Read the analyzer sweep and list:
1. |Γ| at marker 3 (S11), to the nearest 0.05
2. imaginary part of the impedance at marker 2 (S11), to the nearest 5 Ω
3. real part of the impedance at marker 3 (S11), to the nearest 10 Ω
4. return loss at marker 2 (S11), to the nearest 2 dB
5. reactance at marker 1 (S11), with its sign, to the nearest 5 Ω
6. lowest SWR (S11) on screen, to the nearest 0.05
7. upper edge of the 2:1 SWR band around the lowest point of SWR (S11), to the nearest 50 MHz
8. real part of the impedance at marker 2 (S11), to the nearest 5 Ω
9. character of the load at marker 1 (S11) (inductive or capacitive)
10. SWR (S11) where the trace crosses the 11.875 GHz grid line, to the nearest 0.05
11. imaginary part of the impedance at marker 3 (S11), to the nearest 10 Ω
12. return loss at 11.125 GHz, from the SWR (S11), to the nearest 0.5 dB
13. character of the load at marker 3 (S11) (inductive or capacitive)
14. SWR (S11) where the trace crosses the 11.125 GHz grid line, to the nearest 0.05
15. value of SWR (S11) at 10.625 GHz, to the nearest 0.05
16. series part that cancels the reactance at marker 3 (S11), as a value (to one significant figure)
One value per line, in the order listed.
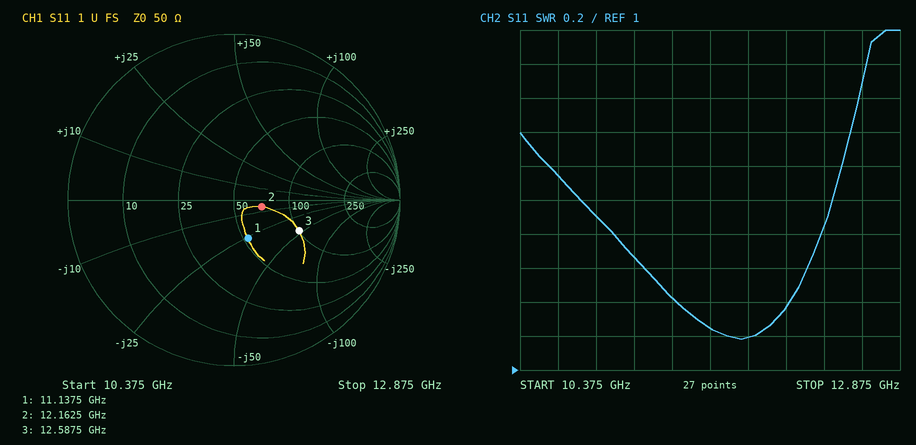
0.45
-5 Ω
100 Ω
16 dB
-25 Ω
1.20
12.45 GHz
70 Ω
capacitive
1.20
-50 Ω
12.0 dB
capacitive
1.65
2.15
600 pH
